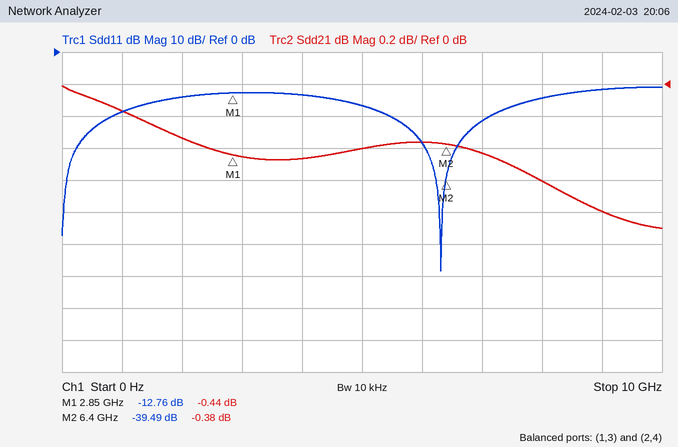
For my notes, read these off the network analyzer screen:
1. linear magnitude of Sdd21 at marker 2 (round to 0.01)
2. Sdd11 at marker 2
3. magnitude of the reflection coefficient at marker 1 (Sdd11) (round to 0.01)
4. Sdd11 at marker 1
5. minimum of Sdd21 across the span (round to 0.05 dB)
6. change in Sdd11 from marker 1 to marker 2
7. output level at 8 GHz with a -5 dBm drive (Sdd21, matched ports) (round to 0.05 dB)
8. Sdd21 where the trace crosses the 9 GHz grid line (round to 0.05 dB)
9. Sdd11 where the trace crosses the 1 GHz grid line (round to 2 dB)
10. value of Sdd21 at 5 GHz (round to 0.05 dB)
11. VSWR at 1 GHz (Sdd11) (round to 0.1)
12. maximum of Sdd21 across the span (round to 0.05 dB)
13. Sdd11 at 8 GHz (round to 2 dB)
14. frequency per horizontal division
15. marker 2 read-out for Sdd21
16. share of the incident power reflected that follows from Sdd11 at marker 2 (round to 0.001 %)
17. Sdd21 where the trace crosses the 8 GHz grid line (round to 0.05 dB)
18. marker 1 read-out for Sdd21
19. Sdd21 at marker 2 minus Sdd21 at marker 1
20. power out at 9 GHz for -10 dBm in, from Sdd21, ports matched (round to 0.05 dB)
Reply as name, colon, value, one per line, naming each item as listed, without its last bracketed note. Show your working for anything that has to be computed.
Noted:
linear magnitude of Sdd21 at marker 2: 10^(-0.38/20) ≈ 0.96
Sdd11 at marker 2: -39.49 dB
magnitude of the reflection coefficient at marker 1 (Sdd11): 10^(-12.76/20) ≈ 0.23
Sdd11 at marker 1: -12.76 dB
minimum of Sdd21 across the span: -0.90 dB
change in Sdd11 from marker 1 to marker 2: -39.49 − (-12.76) = -26.73 dB
output level at 8 GHz with a -5 dBm drive (Sdd21, matched ports): -5 dBm + (-0.60 dB) = -5.60 dBm
Sdd21 where the trace crosses the 9 GHz grid line: -0.80 dB
Sdd11 where the trace crosses the 1 GHz grid line: -18 dB
value of Sdd21 at 5 GHz: -0.40 dB
VSWR at 1 GHz (Sdd11): |Γ| = 10^(-18/20) = 0.1259; VSWR = (1 + 0.1259)/(1 − 0.1259) ≈ 1.3
maximum of Sdd21 across the span: 0.00 dB
Sdd11 at 8 GHz: -14 dB
frequency per horizontal division: 1 GHz
marker 2 read-out for Sdd21: -0.38 dB
share of the incident power reflected that follows from Sdd11 at marker 2: 10^(-39.49/10) ≈ 0.011 %
Sdd21 where the trace crosses the 8 GHz grid line: -0.60 dB
marker 1 read-out for Sdd21: -0.44 dB
Sdd21 at marker 2 minus Sdd21 at marker 1: -0.38 − (-0.44) = 0.06 dB
power out at 9 GHz for -10 dBm in, from Sdd21, ports matched: -10 dBm + (-0.80 dB) = -10.80 dBm
